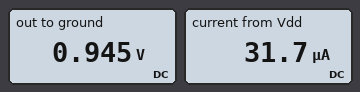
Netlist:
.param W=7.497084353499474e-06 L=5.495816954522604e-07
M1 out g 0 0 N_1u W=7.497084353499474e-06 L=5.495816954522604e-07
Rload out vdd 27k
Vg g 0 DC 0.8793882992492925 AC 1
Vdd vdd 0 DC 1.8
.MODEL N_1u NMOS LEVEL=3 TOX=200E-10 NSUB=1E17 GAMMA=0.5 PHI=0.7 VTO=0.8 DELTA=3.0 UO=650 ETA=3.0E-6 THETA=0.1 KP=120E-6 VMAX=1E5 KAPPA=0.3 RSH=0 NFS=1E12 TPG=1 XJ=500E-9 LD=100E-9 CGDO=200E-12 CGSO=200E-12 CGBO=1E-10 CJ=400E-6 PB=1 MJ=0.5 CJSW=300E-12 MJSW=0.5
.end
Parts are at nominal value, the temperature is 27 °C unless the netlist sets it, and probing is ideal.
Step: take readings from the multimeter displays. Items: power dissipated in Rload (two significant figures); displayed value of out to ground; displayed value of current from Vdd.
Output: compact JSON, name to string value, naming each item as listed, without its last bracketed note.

{"power dissipated in Rload": "27 µW", "displayed value of out to ground": "0.945 V", "displayed value of current from Vdd": "31.7 µA"}
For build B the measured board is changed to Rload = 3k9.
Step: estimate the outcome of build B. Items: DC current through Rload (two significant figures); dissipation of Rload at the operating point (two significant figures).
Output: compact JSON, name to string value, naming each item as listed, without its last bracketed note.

{"DC current through Rload": "34 µA", "dissipation of Rload at the operating point": "4.5 µW"}
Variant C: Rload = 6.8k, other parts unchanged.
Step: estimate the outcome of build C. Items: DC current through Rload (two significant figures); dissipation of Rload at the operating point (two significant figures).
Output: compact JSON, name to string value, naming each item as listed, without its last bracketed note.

{"DC current through Rload": "34 µA", "dissipation of Rload at the operating point": "7.7 µW"}
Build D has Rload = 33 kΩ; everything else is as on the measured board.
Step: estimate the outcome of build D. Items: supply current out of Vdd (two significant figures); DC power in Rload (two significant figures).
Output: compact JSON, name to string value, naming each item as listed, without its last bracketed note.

{"supply current out of Vdd": "31 µA", "DC power in Rload": "32 µW"}
